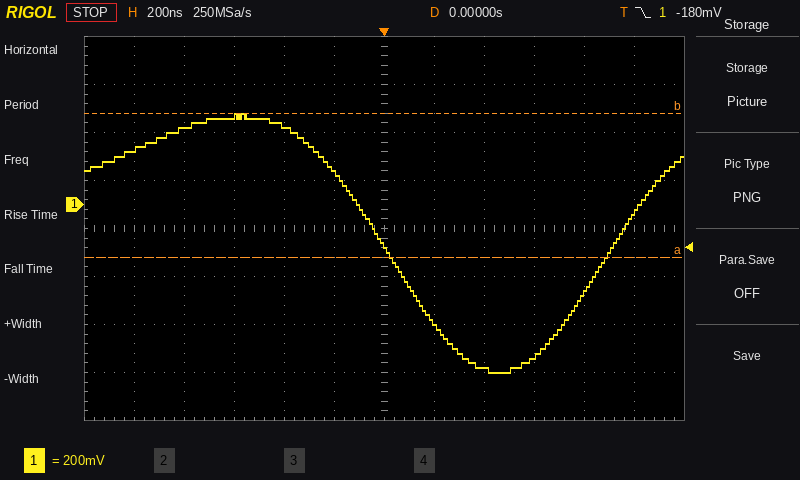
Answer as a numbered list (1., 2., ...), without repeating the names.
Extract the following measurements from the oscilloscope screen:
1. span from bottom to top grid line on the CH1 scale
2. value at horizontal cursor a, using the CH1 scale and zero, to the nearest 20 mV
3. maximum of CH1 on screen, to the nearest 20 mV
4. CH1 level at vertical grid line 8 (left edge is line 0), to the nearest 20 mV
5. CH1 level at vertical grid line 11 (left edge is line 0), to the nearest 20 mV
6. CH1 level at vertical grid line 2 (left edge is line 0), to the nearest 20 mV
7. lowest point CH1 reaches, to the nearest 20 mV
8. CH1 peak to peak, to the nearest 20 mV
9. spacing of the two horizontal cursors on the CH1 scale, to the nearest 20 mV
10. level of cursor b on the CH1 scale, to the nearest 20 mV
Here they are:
1. 1.6 V
2. -220 mV
3. 380 mV
4. -680 mV
5. -40 mV
6. 320 mV
7. -700 mV
8. 1.08 V
9. 600 mV
10. 380 mV
